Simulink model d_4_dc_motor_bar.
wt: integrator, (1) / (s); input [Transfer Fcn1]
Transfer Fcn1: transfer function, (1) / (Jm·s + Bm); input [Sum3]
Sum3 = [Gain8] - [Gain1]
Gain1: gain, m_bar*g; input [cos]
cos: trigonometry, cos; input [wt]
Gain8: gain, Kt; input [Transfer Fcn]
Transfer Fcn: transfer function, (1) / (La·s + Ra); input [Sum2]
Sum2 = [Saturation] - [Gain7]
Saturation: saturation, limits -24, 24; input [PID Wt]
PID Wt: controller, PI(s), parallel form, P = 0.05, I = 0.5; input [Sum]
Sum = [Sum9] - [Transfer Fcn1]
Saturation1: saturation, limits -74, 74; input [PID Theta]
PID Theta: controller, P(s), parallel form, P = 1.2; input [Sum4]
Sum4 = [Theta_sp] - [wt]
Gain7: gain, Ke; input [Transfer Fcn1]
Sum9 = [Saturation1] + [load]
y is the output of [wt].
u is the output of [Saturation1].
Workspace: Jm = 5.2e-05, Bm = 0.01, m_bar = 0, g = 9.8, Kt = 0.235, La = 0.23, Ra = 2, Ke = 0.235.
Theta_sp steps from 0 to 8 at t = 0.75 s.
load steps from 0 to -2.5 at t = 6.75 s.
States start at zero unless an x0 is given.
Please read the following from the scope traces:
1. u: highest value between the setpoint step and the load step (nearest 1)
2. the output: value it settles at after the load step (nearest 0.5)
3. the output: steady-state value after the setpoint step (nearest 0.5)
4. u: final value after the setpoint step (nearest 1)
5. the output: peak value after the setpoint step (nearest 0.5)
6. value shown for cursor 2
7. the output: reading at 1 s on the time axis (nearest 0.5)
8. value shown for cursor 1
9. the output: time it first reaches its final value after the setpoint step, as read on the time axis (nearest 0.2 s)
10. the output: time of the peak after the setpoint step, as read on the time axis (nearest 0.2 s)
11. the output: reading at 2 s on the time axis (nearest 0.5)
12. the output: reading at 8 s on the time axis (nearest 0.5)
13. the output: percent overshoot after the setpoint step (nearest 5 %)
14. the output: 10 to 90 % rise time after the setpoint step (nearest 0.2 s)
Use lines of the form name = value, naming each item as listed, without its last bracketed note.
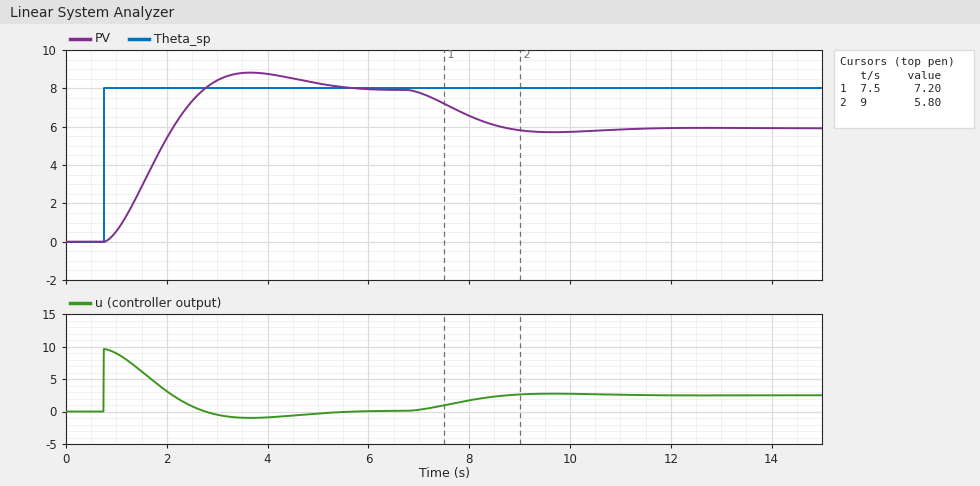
u: highest value between the setpoint step and the load step = 10
the output: value it settles at after the load step = 6.0
the output: steady-state value after the setpoint step = 8.0
u: final value after the setpoint step = 0
the output: peak value after the setpoint step = 9.0
value shown for cursor 2 = 5.80
the output: reading at 1 s on the time axis = 0.5
value shown for cursor 1 = 7.20
the output: time it first reaches its final value after the setpoint step, as read on the time axis = 2.8 s
the output: time of the peak after the setpoint step, as read on the time axis = 3.6 s
the output: reading at 2 s on the time axis = 5.5
the output: reading at 8 s on the time axis = 6.5
the output: percent overshoot after the setpoint step = 10 %
the output: 10 to 90 % rise time after the setpoint step = 1.4 s
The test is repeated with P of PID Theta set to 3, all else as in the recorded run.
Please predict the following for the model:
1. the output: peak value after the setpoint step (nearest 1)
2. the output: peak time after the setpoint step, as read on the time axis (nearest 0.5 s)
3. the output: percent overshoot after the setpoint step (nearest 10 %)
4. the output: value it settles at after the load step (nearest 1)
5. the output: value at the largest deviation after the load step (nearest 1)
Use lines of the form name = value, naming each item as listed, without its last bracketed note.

the output: peak value after the setpoint step = 10
the output: peak time after the setpoint step, as read on the time axis = 2.5 s
the output: percent overshoot after the setpoint step = 20 %
the output: value it settles at after the load step = 7
the output: value at the largest deviation after the load step = 7
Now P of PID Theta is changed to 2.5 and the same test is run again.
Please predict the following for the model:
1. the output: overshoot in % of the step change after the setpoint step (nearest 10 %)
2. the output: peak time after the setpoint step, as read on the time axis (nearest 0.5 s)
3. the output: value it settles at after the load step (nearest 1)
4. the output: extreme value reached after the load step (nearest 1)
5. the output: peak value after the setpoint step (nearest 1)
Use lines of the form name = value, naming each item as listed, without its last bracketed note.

the output: overshoot in % of the step change after the setpoint step = 20 %
the output: peak time after the setpoint step, as read on the time axis = 2.5 s
the output: value it settles at after the load step = 7
the output: extreme value reached after the load step = 7
the output: peak value after the setpoint step = 10
